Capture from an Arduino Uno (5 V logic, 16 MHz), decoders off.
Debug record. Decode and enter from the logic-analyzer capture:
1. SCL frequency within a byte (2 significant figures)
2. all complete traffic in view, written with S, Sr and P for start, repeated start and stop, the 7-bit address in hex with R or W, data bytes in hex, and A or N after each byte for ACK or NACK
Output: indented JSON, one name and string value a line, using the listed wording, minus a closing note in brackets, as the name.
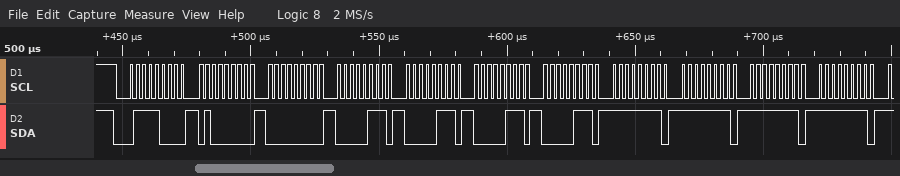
{
  "SCL frequency within a byte": "400 kHz",
  "all complete traffic in view, written with S, Sr and P for start, repeated start and stop, the 7-bit address in hex with R or W, data bytes in hex, and A or N after each byte for ACK or NACK": "S 3CW A 40 A 00 A 07 A 07 A 07 A 07 A FF A FF A FF A FF A"
}
